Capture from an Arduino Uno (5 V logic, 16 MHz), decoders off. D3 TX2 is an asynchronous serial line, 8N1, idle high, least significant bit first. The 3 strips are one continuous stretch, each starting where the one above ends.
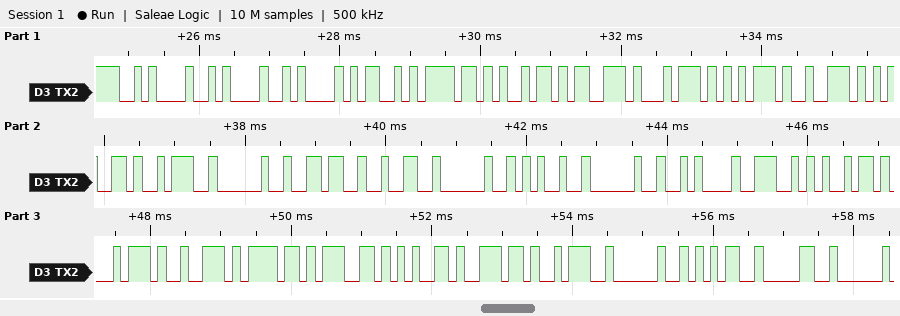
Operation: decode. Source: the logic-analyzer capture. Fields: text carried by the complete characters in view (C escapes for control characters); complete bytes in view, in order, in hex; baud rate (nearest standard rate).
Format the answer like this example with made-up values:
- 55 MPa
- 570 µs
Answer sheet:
- "\n\n\nMoisture: 62 % \nNitrogen: 50"
- 0A 0A 0A 4D 6F 69 73 74 75 72 65 3A 20 36 32 20 25 20 0A 4E 69 74 72 6F 67 65 6E 3A 20 35 30
- 9600 baud
